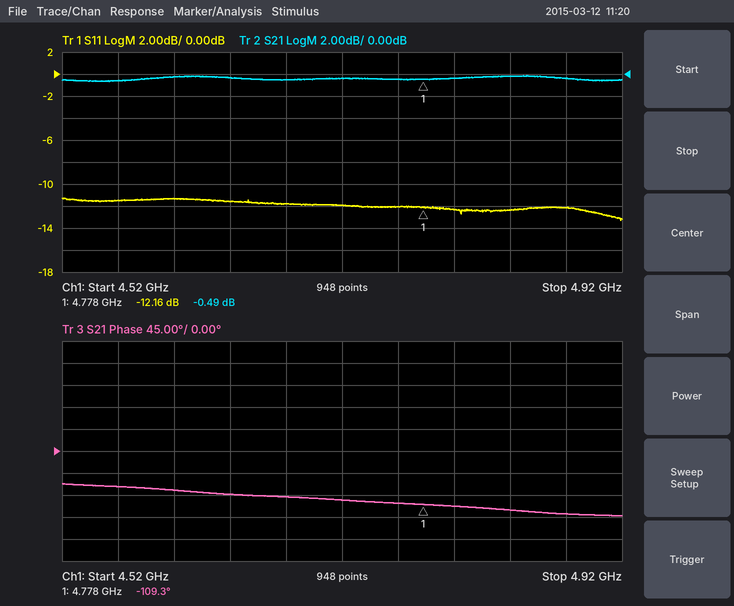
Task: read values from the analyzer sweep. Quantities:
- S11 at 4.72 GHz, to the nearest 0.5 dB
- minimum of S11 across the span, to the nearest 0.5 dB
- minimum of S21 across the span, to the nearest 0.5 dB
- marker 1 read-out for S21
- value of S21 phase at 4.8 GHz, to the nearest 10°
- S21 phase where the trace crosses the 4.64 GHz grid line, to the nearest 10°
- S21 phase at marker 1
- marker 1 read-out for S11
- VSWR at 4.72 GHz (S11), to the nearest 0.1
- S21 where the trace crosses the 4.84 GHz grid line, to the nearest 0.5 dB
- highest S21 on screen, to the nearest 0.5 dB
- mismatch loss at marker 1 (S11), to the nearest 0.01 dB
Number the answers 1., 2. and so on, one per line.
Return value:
1. -12.0 dB
2. -13.5 dB
3. -0.5 dB
4. -0.49 dB
5. -110°
6. -90°
7. -109.3°
8. -12.16 dB
9. 1.7
10. 0.0 dB
11. 0.0 dB
12. 0.27 dB
